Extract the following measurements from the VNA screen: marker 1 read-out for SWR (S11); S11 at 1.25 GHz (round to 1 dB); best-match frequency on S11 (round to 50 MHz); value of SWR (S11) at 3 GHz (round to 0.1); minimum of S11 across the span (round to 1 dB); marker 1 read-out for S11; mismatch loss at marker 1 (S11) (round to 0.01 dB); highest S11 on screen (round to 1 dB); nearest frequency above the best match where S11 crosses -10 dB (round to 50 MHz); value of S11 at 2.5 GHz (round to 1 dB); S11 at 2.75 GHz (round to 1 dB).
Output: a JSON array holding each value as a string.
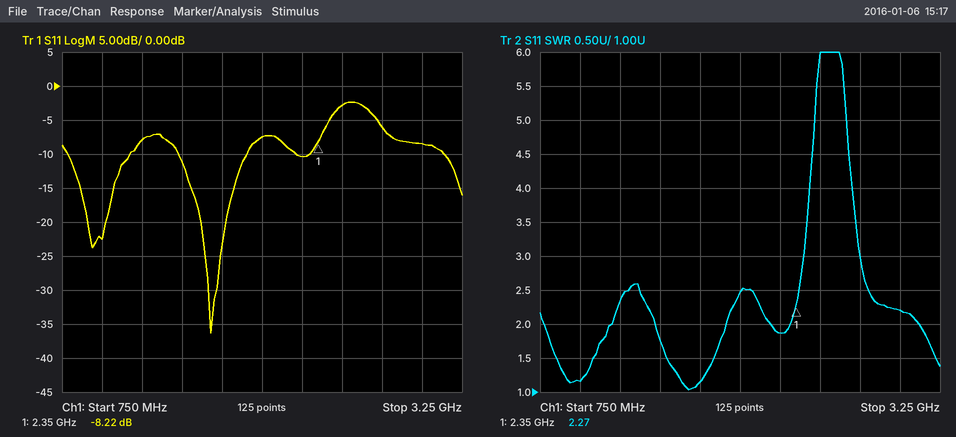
["2.27", "-8 dB", "1.70 GHz", "2.2", "-36 dB", "-8.22 dB", "0.71 dB", "-2 dB", "1.90 GHz", "-3 dB", "-6 dB"]
